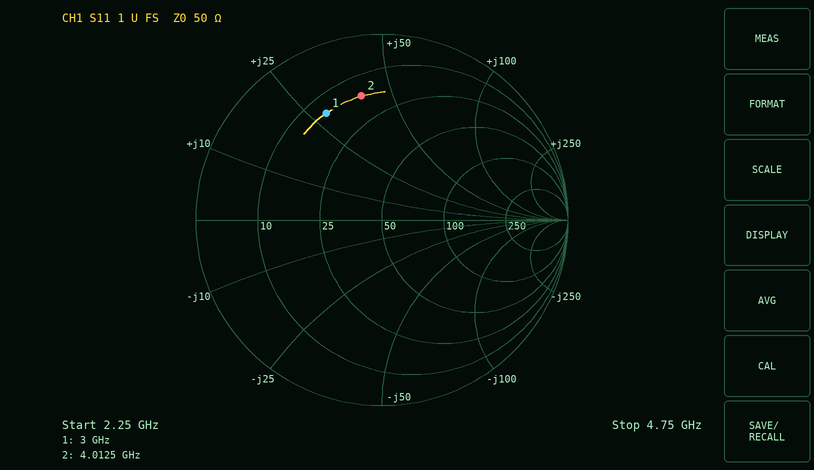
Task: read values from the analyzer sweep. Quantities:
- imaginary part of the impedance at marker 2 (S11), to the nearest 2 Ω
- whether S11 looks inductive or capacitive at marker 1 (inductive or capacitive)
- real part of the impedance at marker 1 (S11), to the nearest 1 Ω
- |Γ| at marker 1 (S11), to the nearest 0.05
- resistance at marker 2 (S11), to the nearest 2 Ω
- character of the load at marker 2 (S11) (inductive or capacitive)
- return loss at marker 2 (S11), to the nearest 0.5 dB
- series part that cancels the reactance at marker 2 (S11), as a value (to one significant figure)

+40 Ω
inductive
14 Ω
0.65
16 Ω
inductive
3.5 dB
1.0 pF
